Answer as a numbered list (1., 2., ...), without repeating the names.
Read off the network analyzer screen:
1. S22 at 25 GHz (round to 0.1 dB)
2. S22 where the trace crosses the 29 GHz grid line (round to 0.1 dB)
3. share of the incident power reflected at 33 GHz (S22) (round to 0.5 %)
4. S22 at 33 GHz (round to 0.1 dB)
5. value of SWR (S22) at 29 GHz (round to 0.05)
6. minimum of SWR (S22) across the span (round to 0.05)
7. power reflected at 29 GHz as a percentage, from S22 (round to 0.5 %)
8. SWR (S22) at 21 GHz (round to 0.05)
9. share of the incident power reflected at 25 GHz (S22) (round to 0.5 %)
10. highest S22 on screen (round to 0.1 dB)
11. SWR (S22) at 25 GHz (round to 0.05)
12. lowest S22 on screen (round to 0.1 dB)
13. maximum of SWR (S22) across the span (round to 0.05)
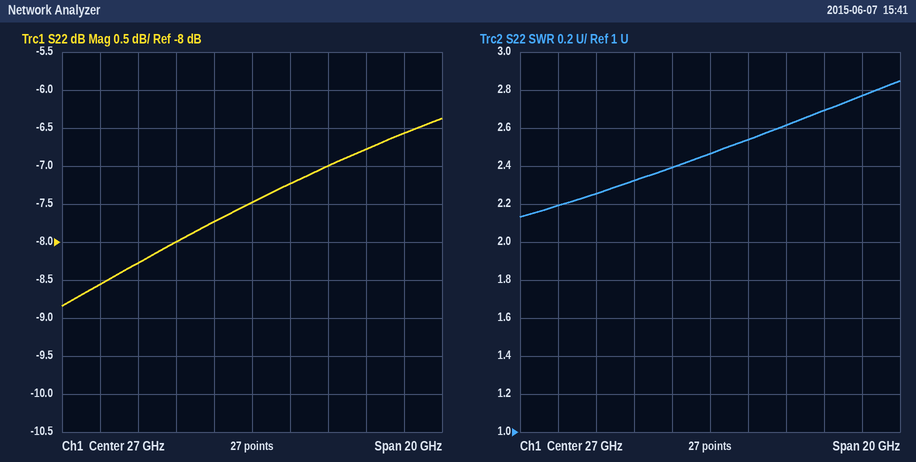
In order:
1. -7.7 dB
2. -7.2 dB
3. 21.0 %
4. -6.8 dB
5. 2.55
6. 2.15
7. 19.0 %
8. 2.25
9. 17.0 %
10. -6.4 dB
11. 2.40
12. -8.8 dB
13. 2.85
